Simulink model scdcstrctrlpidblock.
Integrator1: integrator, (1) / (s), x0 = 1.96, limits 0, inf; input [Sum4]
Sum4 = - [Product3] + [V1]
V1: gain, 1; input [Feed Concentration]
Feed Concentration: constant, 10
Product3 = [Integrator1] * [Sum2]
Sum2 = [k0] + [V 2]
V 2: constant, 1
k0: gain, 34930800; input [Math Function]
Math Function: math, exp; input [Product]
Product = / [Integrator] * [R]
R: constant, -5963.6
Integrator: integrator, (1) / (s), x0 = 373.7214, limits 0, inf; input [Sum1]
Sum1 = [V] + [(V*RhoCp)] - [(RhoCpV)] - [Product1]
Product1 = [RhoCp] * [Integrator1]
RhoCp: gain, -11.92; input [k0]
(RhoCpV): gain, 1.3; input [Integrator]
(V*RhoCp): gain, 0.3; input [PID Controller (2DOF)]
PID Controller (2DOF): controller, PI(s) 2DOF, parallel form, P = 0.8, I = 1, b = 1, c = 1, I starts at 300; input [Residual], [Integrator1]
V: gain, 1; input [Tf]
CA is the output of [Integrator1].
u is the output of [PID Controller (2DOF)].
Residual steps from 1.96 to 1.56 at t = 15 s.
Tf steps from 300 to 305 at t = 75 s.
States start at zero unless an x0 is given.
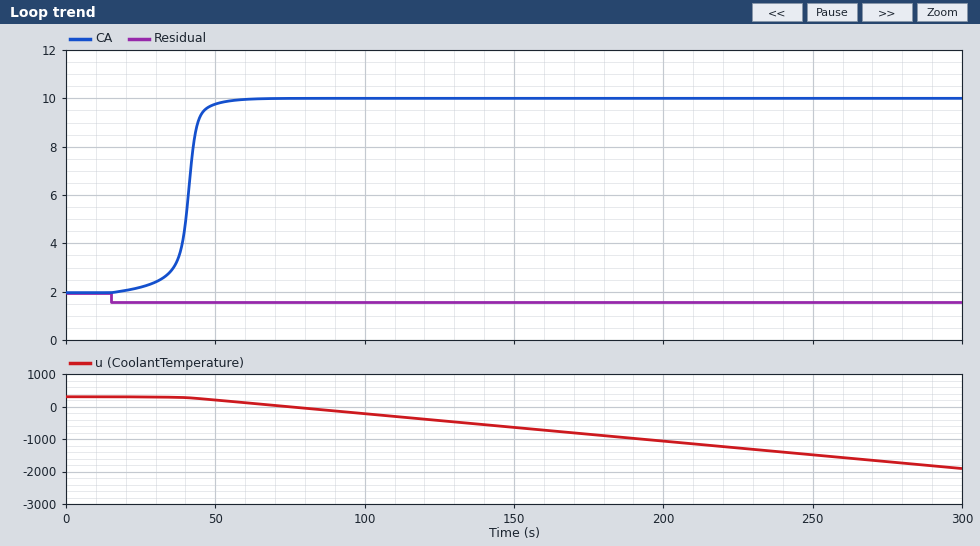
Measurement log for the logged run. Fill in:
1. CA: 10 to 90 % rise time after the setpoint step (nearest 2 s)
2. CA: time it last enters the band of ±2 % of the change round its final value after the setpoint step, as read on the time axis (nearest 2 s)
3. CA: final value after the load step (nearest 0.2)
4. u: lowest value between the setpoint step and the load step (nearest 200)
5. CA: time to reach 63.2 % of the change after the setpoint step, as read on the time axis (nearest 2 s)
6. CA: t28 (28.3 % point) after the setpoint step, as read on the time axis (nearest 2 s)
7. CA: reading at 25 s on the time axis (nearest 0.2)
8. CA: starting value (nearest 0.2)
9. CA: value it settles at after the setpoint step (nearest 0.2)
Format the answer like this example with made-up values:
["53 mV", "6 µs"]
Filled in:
["10 s", "52 s", "10.0", "0", "42 s", "40 s", "2.2", "2.0", "10.0"]
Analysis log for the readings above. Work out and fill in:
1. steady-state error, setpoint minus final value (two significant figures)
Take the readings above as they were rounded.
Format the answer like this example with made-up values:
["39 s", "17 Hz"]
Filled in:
["-8.4"]
